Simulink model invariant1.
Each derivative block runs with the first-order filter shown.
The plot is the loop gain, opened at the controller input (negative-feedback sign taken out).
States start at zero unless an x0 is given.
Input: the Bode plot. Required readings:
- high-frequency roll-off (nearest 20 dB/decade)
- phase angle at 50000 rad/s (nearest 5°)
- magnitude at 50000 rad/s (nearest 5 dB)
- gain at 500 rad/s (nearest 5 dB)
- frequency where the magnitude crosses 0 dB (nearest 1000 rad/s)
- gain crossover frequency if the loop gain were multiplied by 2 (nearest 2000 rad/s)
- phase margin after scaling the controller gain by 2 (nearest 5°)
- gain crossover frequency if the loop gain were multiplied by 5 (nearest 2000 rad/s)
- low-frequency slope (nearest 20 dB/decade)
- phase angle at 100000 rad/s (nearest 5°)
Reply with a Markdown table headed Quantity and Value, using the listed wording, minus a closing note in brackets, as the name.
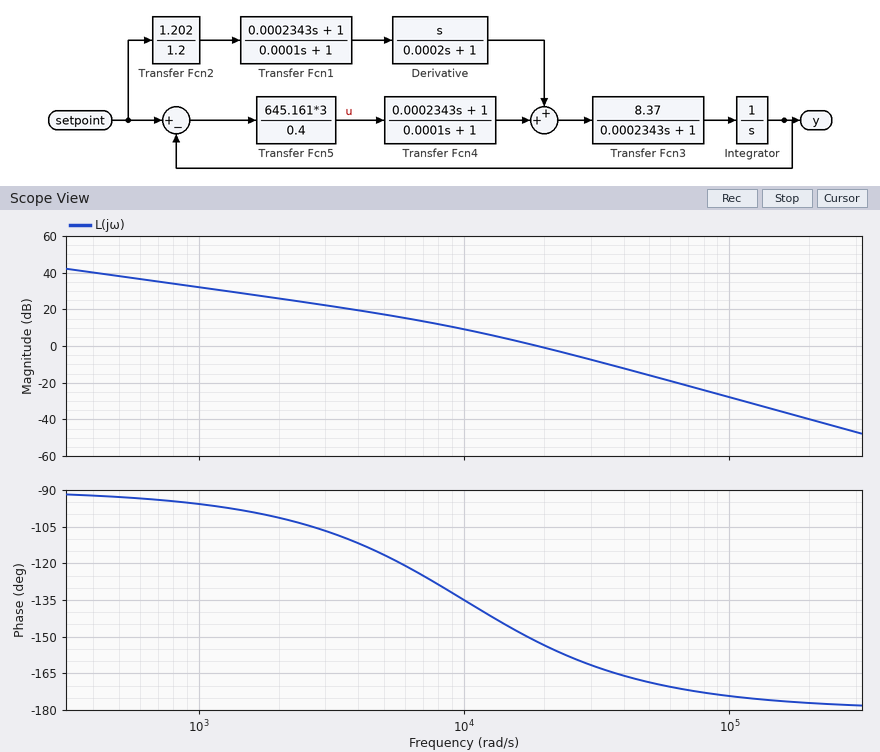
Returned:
| Quantity | Value |
|---|---|
| high-frequency roll-off | -40 dB/decade |
| phase angle at 50000 rad/s | -170° |
| magnitude at 50000 rad/s | -15 dB |
| gain at 500 rad/s | 40 dB |
| frequency where the magnitude crosses 0 dB | 19000 rad/s |
| gain crossover frequency if the loop gain were multiplied by 2 | 28000 rad/s |
| phase margin after scaling the controller gain by 2 | 20° |
| gain crossover frequency if the loop gain were multiplied by 5 | 44000 rad/s |
| low-frequency slope | -20 dB/decade |
| phase angle at 100000 rad/s | -175° |
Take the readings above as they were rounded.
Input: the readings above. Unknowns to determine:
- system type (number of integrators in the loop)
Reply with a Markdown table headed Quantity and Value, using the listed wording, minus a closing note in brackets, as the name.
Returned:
| Quantity | Value |
|---|---|
| system type | 1 |
